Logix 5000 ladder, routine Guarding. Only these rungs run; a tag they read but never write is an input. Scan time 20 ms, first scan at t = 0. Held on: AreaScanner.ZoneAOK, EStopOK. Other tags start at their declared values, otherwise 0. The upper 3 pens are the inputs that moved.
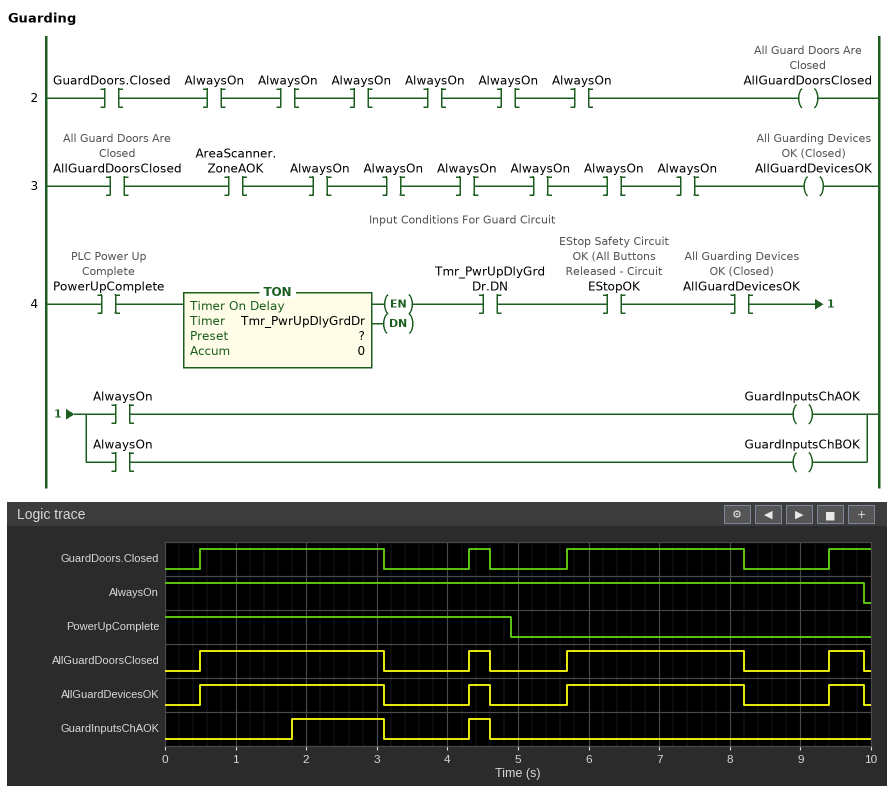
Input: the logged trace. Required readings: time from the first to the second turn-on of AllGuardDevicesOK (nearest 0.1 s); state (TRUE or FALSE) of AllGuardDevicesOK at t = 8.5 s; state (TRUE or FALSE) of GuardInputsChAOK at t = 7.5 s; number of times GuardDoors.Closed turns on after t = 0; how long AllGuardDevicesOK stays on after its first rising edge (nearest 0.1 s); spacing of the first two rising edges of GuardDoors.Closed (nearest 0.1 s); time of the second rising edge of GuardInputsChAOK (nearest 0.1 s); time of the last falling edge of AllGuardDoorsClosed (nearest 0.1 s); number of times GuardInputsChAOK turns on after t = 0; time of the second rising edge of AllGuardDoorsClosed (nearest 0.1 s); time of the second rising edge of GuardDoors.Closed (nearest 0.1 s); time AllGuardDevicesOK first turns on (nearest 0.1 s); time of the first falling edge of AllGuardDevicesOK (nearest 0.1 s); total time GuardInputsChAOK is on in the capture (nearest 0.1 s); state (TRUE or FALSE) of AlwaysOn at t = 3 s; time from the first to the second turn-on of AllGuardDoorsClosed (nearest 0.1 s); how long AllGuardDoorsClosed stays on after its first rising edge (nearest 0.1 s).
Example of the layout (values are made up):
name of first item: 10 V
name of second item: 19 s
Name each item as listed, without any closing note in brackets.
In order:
time from the first to the second turn-on of AllGuardDevicesOK: 3.8 s
state (TRUE or FALSE) of AllGuardDevicesOK at t = 8.5 s: FALSE
state (TRUE or FALSE) of GuardInputsChAOK at t = 7.5 s: FALSE
number of times GuardDoors.Closed turns on after t = 0: 4
how long AllGuardDevicesOK stays on after its first rising edge: 2.6 s
spacing of the first two rising edges of GuardDoors.Closed: 3.8 s
time of the second rising edge of GuardInputsChAOK: 4.3 s
time of the last falling edge of AllGuardDoorsClosed: 9.9 s
number of times GuardInputsChAOK turns on after t = 0: 2
time of the second rising edge of AllGuardDoorsClosed: 4.3 s
time of the second rising edge of GuardDoors.Closed: 4.3 s
time AllGuardDevicesOK first turns on: 0.5 s
time of the first falling edge of AllGuardDevicesOK: 3.1 s
total time GuardInputsChAOK is on in the capture: 1.6 s
state (TRUE or FALSE) of AlwaysOn at t = 3 s: TRUE
time from the first to the second turn-on of AllGuardDoorsClosed: 3.8 s
how long AllGuardDoorsClosed stays on after its first rising edge: 2.6 s
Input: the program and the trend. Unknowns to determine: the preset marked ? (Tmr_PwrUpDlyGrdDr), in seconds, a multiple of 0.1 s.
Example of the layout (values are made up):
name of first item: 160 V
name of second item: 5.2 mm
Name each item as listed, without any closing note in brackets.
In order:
the preset marked ? (Tmr_PwrUpDlyGrdDr), in seconds, a multiple of 0.1 s: 1.8 s
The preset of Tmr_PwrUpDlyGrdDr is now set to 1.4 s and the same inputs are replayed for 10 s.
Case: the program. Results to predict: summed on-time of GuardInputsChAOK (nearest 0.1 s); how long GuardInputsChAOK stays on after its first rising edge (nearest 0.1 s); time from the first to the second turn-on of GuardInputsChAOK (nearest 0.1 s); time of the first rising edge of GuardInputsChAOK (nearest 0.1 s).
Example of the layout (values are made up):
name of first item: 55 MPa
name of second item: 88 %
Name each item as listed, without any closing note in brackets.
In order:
summed on-time of GuardInputsChAOK: 2.0 s
how long GuardInputsChAOK stays on after its first rising edge: 1.7 s
time from the first to the second turn-on of GuardInputsChAOK: 2.9 s
time of the first rising edge of GuardInputsChAOK: 1.4 s
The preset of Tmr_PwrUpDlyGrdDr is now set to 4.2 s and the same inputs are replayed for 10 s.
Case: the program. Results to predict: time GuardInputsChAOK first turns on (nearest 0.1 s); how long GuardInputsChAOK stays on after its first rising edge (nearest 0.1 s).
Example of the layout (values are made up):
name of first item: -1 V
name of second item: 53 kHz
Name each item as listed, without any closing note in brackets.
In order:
time GuardInputsChAOK first turns on: 4.3 s
how long GuardInputsChAOK stays on after its first rising edge: 0.3 s
